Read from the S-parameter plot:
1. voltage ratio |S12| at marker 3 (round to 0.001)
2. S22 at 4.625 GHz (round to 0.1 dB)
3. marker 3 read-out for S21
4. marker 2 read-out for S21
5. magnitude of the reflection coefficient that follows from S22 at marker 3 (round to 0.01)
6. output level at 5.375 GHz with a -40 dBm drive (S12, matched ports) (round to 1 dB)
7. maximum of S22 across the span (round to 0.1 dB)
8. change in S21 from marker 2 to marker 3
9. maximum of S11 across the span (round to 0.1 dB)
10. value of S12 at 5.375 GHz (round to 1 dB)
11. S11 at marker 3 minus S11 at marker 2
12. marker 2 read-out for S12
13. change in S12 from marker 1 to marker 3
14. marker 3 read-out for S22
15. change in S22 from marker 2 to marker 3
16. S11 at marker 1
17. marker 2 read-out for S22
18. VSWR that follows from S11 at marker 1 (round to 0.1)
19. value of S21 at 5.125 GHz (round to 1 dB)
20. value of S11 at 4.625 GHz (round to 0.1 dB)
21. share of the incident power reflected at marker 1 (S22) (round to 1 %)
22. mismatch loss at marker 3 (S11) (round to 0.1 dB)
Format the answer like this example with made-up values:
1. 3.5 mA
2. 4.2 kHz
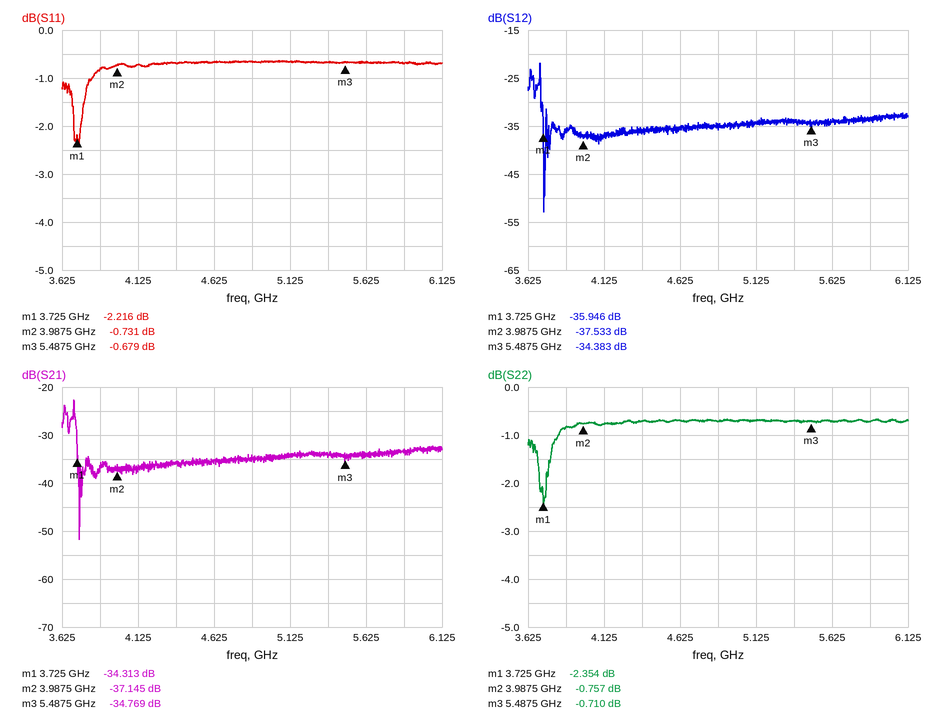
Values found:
1. 0.019
2. -0.7 dB
3. -34.769 dB
4. -37.145 dB
5. 0.92
6. -74 dBm
7. -0.7 dB
8. 2.376 dB
9. -0.6 dB
10. -34 dB
11. 0.052 dB
12. -37.533 dB
13. 1.563 dB
14. -0.710 dB
15. 0.047 dB
16. -2.216 dB
17. -0.757 dB
18. 7.9
19. -34 dB
20. -0.7 dB
21. 58 %
22. 8.4 dB
